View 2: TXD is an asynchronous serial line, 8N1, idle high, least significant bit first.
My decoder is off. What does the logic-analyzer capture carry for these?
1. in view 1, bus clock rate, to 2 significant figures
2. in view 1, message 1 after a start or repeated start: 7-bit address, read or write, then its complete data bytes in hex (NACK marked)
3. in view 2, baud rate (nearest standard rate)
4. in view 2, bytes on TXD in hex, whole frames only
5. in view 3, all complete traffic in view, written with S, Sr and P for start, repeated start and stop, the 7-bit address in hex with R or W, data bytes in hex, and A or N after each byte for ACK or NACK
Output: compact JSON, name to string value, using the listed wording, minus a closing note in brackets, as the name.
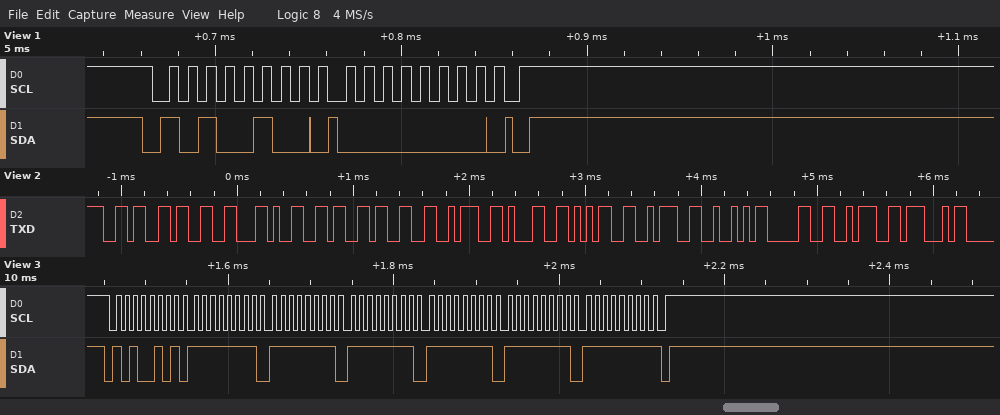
{"in view 1, bus clock rate, to 2 significant figures": "100 kHz", "in view 1, message 1 after a start or repeated start: 7-bit address, read or write, then its complete data bytes in hex": "0x52 write: 00", "in view 2, baud rate": "19200 baud", "in view 2, bytes on TXD in hex, whole frames only": "0x36 0x33 0x2C 0x36 0x33 0x3A 0x31 0x35 0x3A 0x52 0x30 0x3A 0x47", "in view 3, all complete traffic in view, written with S, Sr and P for start, repeated start and stop, the 7-bit address in hex with R or W, data bytes in hex, and A or N after each byte for ACK or NACK": "S 52R A FF A FF A FF A FF A FF A FF N P"}
